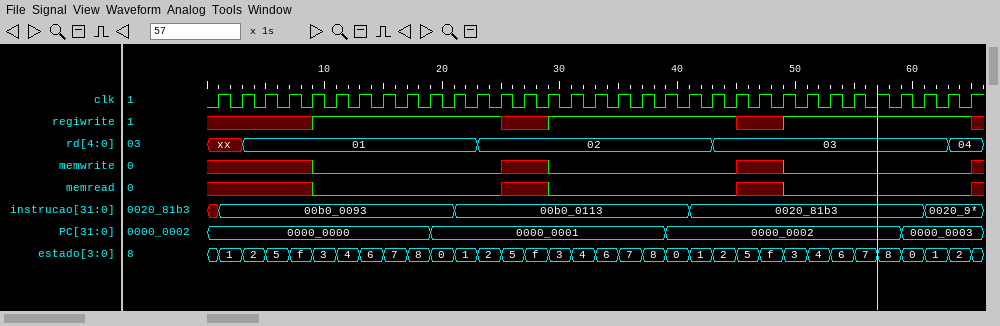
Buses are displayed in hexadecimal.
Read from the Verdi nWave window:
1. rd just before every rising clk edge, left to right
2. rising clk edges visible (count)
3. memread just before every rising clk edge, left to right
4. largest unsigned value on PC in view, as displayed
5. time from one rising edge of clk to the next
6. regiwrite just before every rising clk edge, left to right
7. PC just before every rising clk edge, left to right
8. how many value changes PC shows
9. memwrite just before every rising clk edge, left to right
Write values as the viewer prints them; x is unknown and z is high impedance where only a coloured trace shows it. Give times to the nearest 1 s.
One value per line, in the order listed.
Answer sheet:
xx, xx, 01, 01, 01, 01, 01, 01, 01, 01, 01, 01, 02, 02, 02, 02, 02, 02, 02, 02, 02, 02, 03, 03, 03, 03, 03, 03, 03, 03, 03, 03, 04
33
x x x x x 0 0 0 0 0 0 0 0 x x 0 0 0 0 0 0 0 0 x x 0 0 0 0 0 0 0 0
0000_0003
2 s
x x x x x 1 1 1 1 1 1 1 1 x x 1 1 1 1 1 1 1 1 x x 1 1 1 1 1 1 1 1
0000_0000, 0000_0000, 0000_0000, 0000_0000, 0000_0000, 0000_0000, 0000_0000, 0000_0000, 0000_0000, 0000_0000, 0000_0001, 0000_0001, 0000_0001, 0000_0001, 0000_0001, 0000_0001, 0000_0001, 0000_0001, 0000_0001, 0000_0001, 0000_0002, 0000_0002, 0000_0002, 0000_0002, 0000_0002, 0000_0002, 0000_0002, 0000_0002, 0000_0002, 0000_0002, 0000_0003, 0000_0003, 0000_0003
3
x x x x x 0 0 0 0 0 0 0 0 x x 0 0 0 0 0 0 0 0 x x 0 0 0 0 0 0 0 0
